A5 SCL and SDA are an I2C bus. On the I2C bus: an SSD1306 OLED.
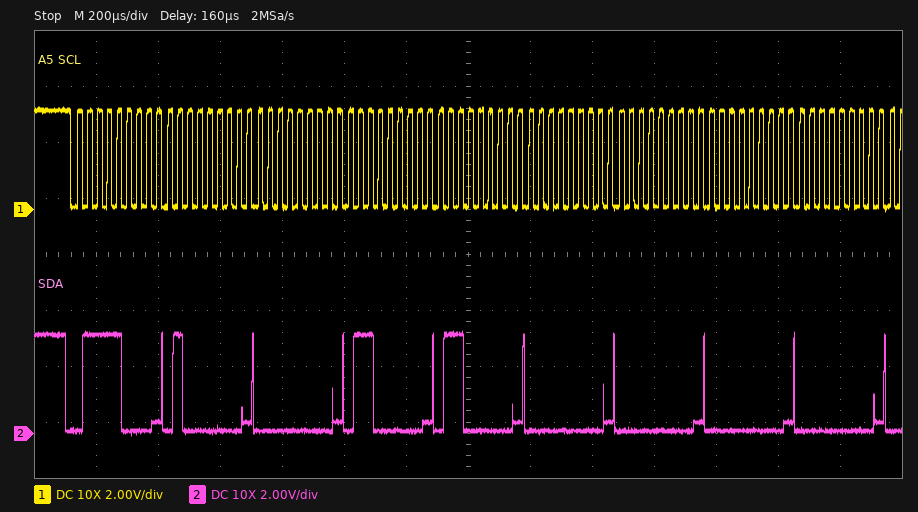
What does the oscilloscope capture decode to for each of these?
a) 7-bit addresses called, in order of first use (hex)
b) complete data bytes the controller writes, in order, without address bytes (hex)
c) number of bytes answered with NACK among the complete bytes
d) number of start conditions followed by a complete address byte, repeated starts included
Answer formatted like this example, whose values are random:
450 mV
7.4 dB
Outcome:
0x3C
40 00 60 60 00 00 00 00
0
1
